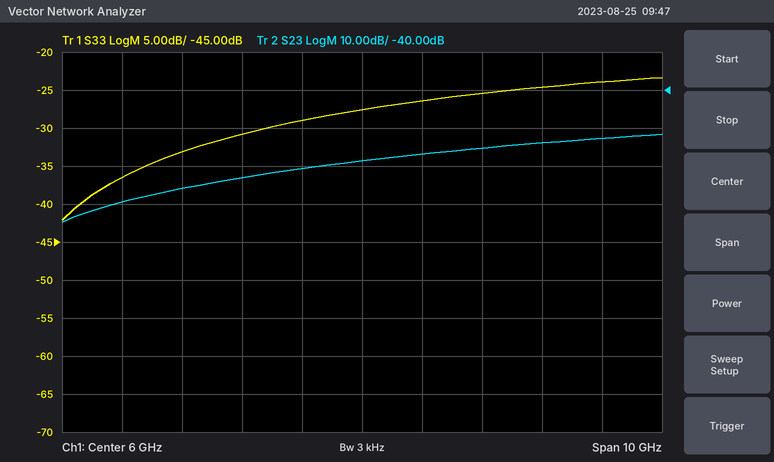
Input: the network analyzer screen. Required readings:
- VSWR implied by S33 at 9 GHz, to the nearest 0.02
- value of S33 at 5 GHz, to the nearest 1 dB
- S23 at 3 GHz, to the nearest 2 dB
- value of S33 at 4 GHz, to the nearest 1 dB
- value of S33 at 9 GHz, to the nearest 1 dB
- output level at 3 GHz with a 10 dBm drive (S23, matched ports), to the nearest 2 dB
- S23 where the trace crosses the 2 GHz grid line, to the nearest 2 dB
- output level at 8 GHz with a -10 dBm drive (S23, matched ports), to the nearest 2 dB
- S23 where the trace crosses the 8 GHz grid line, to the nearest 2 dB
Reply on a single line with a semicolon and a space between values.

1.12; -29 dB; -66 dB; -31 dB; -25 dB; -56 dBm; -70 dB; -66 dBm; -56 dB
